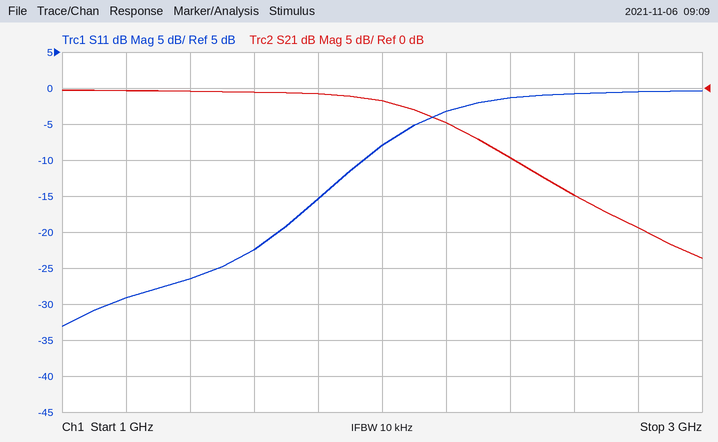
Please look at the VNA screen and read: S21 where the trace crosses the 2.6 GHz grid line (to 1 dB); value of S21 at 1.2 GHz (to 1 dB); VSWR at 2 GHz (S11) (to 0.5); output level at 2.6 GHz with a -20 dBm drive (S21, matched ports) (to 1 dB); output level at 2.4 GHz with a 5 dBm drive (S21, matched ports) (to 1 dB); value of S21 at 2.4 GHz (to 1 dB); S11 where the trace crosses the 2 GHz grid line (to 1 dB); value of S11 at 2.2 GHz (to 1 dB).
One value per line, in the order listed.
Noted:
-15 dB
0 dB
2.5
-35 dBm
-5 dBm
-10 dB
-8 dB
-3 dB
